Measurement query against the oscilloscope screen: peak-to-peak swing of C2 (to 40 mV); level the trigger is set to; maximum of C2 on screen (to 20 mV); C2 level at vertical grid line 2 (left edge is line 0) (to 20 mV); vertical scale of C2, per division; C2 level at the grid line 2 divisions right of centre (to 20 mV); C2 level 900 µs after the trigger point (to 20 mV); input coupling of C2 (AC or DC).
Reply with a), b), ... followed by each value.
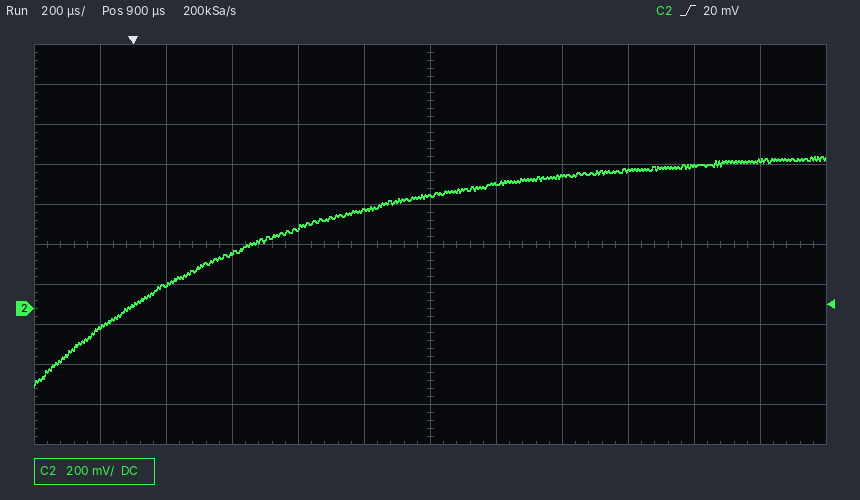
a) 1.16 V
b) 20 mV
c) 760 mV
d) 120 mV
e) 200 mV
f) 660 mV
g) 560 mV
h) DC
